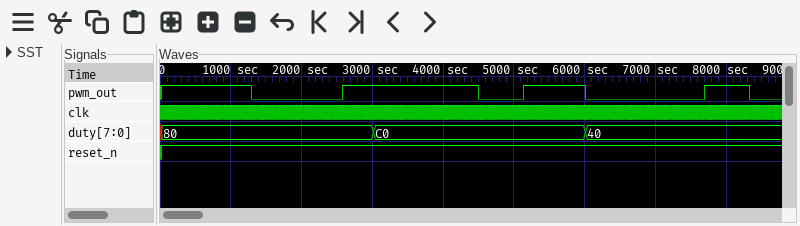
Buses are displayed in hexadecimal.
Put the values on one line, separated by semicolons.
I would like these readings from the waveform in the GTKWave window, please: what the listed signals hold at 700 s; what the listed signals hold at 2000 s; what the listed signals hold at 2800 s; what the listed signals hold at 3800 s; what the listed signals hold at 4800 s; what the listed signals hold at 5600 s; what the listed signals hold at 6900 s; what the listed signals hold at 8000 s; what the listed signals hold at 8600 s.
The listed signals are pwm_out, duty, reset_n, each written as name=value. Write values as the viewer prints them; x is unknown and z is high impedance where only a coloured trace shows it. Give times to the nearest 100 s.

pwm_out=1, duty=80, reset_n=1; pwm_out=0, duty=80, reset_n=1; pwm_out=1, duty=80, reset_n=1; pwm_out=1, duty=C0, reset_n=1; pwm_out=0, duty=C0, reset_n=1; pwm_out=1, duty=C0, reset_n=1; pwm_out=0, duty=40, reset_n=1; pwm_out=1, duty=40, reset_n=1; pwm_out=0, duty=40, reset_n=1
